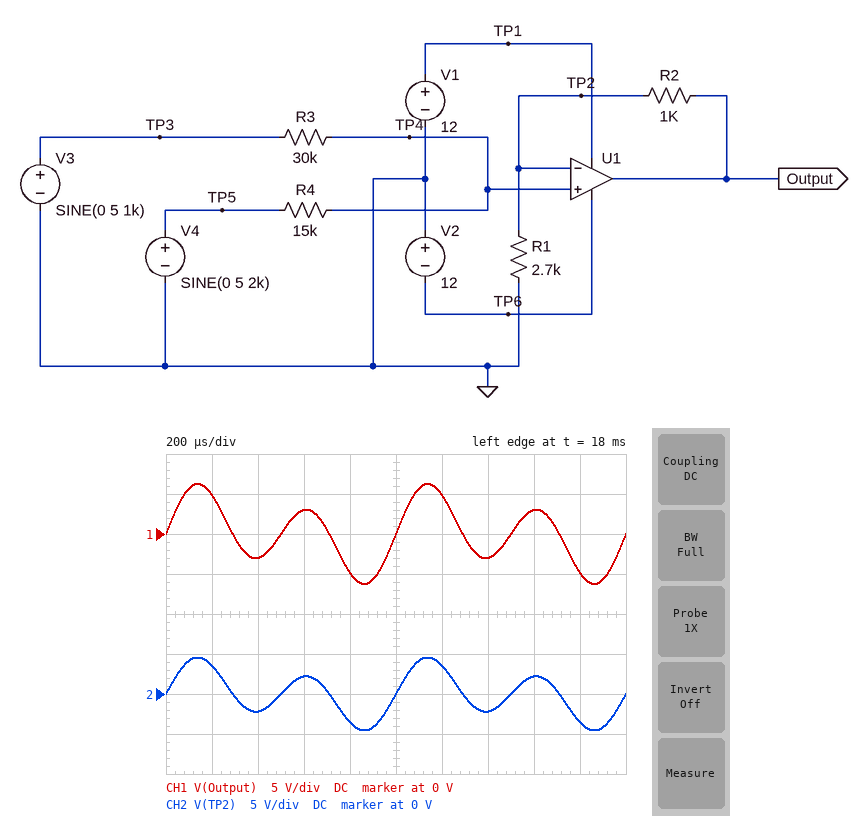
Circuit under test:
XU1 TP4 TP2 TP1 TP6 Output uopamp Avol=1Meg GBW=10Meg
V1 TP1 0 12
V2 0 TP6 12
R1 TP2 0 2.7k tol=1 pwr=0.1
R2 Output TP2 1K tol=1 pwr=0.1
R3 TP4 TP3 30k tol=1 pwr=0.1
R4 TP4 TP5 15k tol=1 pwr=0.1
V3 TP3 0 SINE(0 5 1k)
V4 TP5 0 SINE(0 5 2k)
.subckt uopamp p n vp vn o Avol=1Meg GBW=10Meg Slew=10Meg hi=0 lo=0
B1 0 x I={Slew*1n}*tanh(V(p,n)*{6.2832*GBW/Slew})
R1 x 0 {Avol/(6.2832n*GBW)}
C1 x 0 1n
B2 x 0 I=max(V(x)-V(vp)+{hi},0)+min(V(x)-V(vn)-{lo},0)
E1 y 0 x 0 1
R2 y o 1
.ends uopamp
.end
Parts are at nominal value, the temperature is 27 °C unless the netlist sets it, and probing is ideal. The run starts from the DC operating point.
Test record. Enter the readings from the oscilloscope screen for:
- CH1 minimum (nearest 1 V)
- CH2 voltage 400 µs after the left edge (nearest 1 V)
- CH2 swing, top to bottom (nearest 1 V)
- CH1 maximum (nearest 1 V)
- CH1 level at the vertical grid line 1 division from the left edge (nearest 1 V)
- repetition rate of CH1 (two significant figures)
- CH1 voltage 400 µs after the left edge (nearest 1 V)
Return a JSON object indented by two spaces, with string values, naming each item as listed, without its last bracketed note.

{
  "CH1 minimum": "-6 V",
  "CH2 voltage 400 µs after the left edge": "-2 V",
  "CH2 swing, top to bottom": "9 V",
  "CH1 maximum": "6 V",
  "CH1 level at the vertical grid line 1 division from the left edge": "5 V",
  "repetition rate of CH1": "2.0 kHz",
  "CH1 voltage 400 µs after the left edge": "-3 V"
}
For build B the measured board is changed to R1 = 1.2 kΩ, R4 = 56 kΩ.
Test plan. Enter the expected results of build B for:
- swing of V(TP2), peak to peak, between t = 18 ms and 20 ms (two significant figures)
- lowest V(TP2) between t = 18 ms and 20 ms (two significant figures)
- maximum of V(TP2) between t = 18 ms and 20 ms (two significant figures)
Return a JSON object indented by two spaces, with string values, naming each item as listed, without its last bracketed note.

{
  "swing of V(TP2), peak to peak, between t = 18 ms and 20 ms": "8.7 V",
  "lowest V(TP2) between t = 18 ms and 20 ms": "-4.3 V",
  "maximum of V(TP2) between t = 18 ms and 20 ms": "4.3 V"
}
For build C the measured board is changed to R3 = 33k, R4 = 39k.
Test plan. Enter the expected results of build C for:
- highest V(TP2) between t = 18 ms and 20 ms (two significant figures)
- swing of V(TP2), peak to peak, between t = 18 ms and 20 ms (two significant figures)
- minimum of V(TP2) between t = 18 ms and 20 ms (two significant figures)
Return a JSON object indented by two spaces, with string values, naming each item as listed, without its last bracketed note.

{
  "highest V(TP2) between t = 18 ms and 20 ms": "4.4 V",
  "swing of V(TP2), peak to peak, between t = 18 ms and 20 ms": "8.7 V",
  "minimum of V(TP2) between t = 18 ms and 20 ms": "-4.4 V"
}
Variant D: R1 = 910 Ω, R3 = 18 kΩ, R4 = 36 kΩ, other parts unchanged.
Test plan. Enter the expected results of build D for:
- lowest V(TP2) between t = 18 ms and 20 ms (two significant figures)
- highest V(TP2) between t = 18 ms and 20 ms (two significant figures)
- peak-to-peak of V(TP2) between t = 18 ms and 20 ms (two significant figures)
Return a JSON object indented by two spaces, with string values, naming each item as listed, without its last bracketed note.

{
  "lowest V(TP2) between t = 18 ms and 20 ms": "-4.3 V",
  "highest V(TP2) between t = 18 ms and 20 ms": "4.3 V",
  "peak-to-peak of V(TP2) between t = 18 ms and 20 ms": "8.7 V"
}
